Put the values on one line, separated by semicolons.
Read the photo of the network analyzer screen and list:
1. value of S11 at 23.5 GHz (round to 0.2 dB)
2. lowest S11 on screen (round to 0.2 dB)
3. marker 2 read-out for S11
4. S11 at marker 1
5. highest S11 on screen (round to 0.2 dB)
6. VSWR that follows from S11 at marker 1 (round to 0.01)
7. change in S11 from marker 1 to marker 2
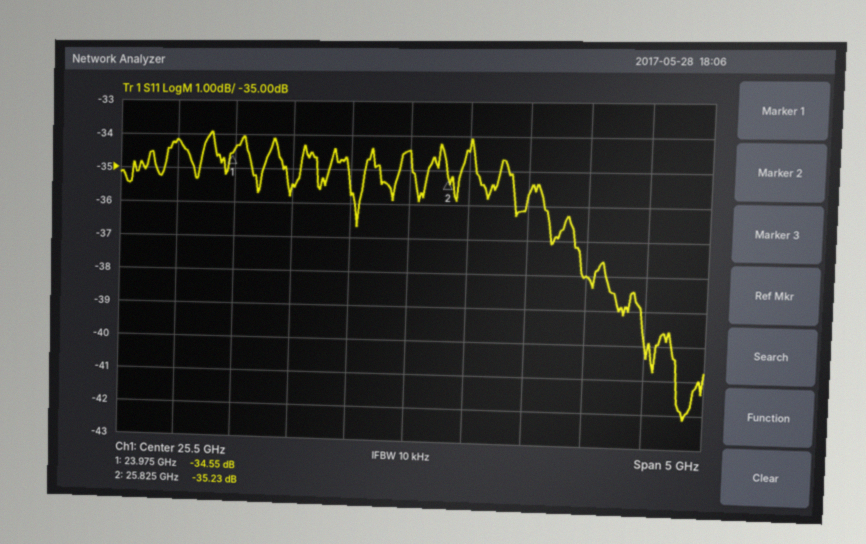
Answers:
-34.2 dB; -42.2 dB; -35.23 dB; -34.55 dB; -34.0 dB; 1.04; -0.68 dB
